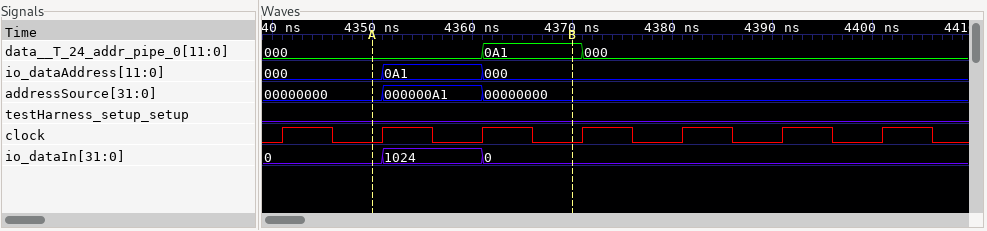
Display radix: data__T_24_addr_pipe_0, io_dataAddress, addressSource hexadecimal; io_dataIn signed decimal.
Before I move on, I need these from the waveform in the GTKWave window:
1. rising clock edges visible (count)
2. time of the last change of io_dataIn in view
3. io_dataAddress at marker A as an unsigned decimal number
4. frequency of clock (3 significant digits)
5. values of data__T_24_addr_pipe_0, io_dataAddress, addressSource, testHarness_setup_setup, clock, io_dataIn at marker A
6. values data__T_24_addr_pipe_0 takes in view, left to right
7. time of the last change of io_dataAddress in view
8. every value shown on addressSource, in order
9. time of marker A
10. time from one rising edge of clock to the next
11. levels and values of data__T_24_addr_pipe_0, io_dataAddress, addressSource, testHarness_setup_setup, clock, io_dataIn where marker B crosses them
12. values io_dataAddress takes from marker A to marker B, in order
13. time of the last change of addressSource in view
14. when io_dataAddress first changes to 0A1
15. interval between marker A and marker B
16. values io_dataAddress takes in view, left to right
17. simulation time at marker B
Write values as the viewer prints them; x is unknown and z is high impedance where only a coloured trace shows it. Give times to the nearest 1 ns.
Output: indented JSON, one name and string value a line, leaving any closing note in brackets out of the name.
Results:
{
  "rising clock edges visible": "7",
  "time of the last change of io_dataIn in view": "4361 ns",
  "io_dataAddress at marker A as an unsigned decimal number": "0",
  "frequency of clock": "100 MHz",
  "values of data__T_24_addr_pipe_0, io_dataAddress, addressSource, testHarness_setup_setup, clock, io_dataIn at marker A": "data__T_24_addr_pipe_0=000, io_dataAddress=000, addressSource=00000000, testHarness_setup_setup=0, clock=0, io_dataIn=0",
  "values data__T_24_addr_pipe_0 takes in view, left to right": "000, 0A1, 000",
  "time of the last change of io_dataAddress in view": "4361 ns",
  "every value shown on addressSource, in order": "00000000, 000000A1, 00000000",
  "time of marker A": "4350 ns",
  "time from one rising edge of clock to the next": "10 ns",
  "levels and values of data__T_24_addr_pipe_0, io_dataAddress, addressSource, testHarness_setup_setup, clock, io_dataIn where marker B crosses them": "data__T_24_addr_pipe_0=0A1, io_dataAddress=000, addressSource=00000000, testHarness_setup_setup=0, clock=0, io_dataIn=0",
  "values io_dataAddress takes from marker A to marker B, in order": "000, 0A1, 000",
  "time of the last change of addressSource in view": "4361 ns",
  "when io_dataAddress first changes to 0A1": "4351 ns",
  "interval between marker A and marker B": "20 ns",
  "values io_dataAddress takes in view, left to right": "000, 0A1, 000",
  "simulation time at marker B": "4370 ns"
}
